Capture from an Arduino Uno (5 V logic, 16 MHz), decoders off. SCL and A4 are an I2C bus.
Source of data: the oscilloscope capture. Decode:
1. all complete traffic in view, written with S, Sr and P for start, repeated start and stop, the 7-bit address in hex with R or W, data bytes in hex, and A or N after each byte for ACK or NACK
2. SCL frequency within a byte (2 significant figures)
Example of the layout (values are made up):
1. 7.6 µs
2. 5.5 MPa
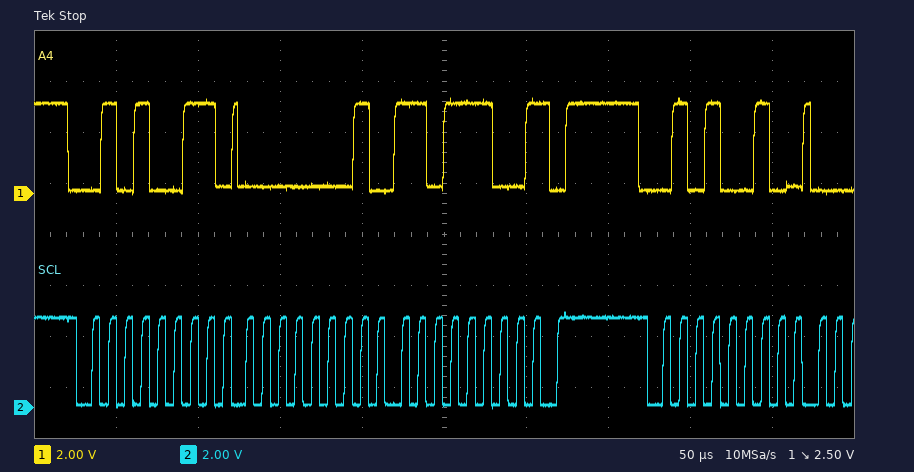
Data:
1. S 29R A 01 A DC N P S 29W A
2. 100 kHz
